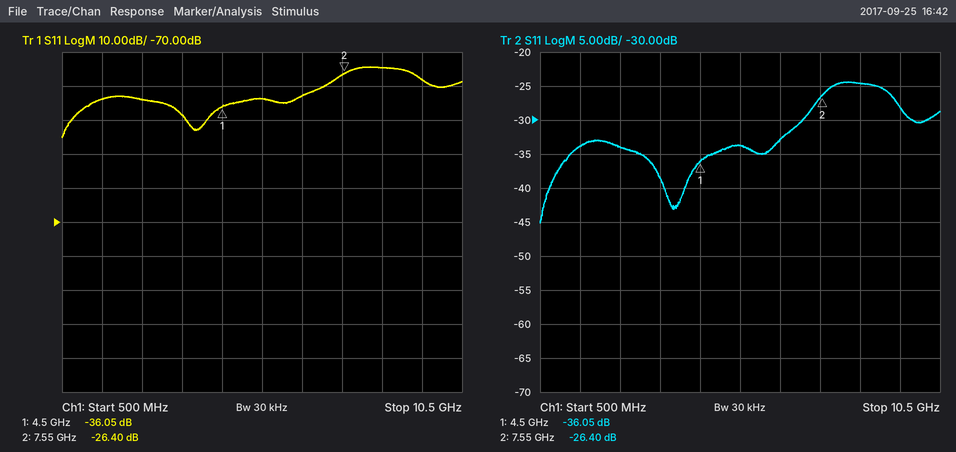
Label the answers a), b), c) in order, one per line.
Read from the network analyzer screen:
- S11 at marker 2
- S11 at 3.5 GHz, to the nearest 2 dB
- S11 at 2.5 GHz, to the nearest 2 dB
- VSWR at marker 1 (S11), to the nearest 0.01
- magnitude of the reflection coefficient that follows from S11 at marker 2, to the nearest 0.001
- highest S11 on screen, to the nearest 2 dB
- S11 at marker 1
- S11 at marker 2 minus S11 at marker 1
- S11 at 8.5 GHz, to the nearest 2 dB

a) -26.40 dB
b) -38 dB
c) -34 dB
d) 1.03
e) 0.048
f) -24 dB
g) -36.05 dB
h) 9.65 dB
i) -24 dB
